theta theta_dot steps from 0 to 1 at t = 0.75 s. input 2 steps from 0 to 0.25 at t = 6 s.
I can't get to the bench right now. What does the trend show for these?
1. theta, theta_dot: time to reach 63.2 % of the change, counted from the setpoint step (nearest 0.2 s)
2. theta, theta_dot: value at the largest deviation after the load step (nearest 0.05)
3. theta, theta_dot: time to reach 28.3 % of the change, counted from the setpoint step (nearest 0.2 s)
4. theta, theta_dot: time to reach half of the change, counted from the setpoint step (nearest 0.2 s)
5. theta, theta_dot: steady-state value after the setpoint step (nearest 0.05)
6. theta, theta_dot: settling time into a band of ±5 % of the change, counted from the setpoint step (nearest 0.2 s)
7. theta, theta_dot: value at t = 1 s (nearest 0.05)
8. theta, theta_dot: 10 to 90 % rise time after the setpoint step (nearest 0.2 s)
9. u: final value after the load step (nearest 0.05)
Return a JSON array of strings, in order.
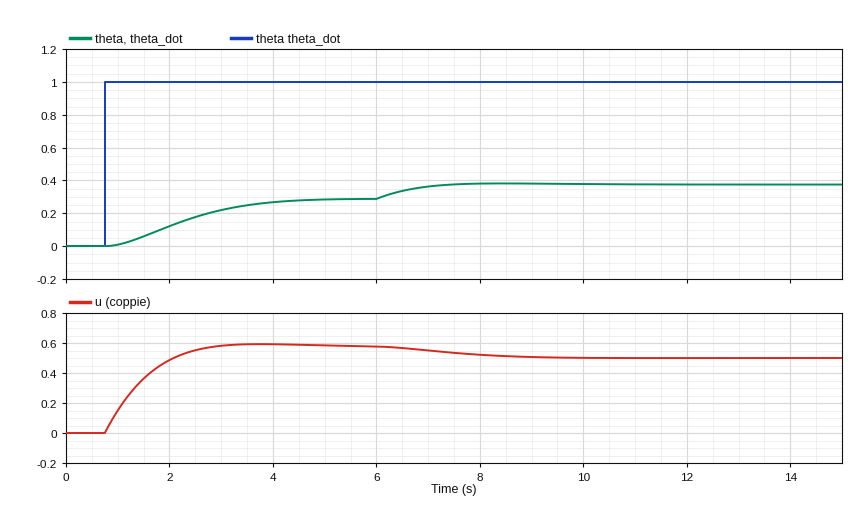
["1.8 s", "0.40", "1.0 s", "1.4 s", "0.30", "3.4 s", "0.00", "2.4 s", "0.50"]
